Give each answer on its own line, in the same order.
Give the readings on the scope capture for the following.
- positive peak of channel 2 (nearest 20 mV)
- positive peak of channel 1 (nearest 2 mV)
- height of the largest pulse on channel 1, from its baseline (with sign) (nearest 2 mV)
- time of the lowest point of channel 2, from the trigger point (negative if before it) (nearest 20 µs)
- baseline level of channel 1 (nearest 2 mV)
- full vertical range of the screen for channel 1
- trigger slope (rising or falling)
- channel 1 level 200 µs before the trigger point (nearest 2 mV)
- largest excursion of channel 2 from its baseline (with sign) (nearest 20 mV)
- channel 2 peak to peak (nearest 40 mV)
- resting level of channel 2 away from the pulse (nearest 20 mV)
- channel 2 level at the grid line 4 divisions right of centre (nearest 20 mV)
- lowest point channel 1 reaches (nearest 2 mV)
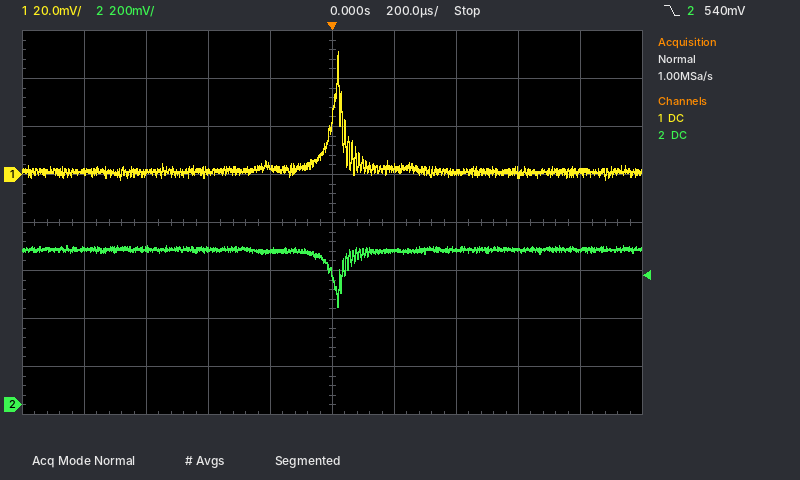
660 mV
52 mV
+50 mV
+20 µs
2 mV
160 mV
falling
4 mV
-240 mV
240 mV
640 mV
640 mV
-2 mV
